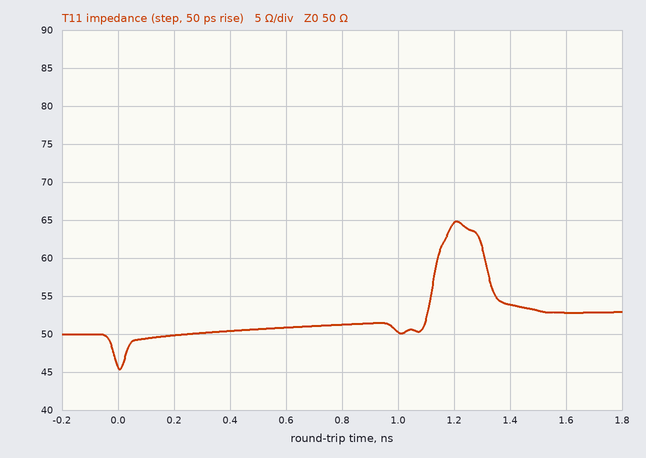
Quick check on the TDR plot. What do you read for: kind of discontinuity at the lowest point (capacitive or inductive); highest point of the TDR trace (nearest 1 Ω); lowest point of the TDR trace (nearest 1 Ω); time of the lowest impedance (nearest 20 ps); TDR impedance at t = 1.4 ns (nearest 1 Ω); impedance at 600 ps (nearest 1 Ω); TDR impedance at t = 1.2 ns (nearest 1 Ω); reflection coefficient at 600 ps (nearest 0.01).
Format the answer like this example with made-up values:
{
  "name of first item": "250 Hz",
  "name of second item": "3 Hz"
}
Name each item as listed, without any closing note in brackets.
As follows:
{
  "kind of discontinuity at the lowest point": "capacitive",
  "highest point of the TDR trace": "65 Ω",
  "lowest point of the TDR trace": "45 Ω",
  "time of the lowest impedance": "0 ps",
  "TDR impedance at t = 1.4 ns": "54 Ω",
  "impedance at 600 ps": "51 Ω",
  "TDR impedance at t = 1.2 ns": "65 Ω",
  "reflection coefficient at 600 ps": "+0.01"
}
